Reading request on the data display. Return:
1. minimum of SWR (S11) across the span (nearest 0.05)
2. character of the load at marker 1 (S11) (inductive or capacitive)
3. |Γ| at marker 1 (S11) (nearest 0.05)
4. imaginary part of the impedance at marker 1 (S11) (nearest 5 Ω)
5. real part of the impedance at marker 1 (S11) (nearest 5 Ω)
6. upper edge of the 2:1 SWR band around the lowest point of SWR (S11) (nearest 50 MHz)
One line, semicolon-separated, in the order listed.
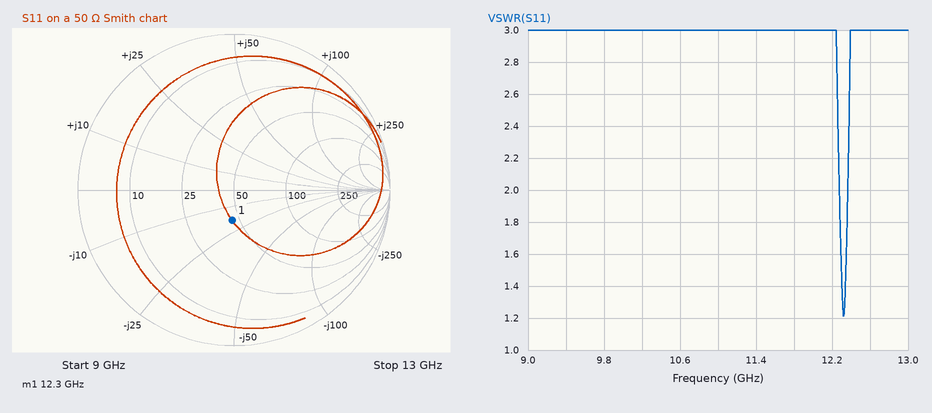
1.20; capacitive; 0.20; -20 Ω; 45 Ω; 12.35 GHz
